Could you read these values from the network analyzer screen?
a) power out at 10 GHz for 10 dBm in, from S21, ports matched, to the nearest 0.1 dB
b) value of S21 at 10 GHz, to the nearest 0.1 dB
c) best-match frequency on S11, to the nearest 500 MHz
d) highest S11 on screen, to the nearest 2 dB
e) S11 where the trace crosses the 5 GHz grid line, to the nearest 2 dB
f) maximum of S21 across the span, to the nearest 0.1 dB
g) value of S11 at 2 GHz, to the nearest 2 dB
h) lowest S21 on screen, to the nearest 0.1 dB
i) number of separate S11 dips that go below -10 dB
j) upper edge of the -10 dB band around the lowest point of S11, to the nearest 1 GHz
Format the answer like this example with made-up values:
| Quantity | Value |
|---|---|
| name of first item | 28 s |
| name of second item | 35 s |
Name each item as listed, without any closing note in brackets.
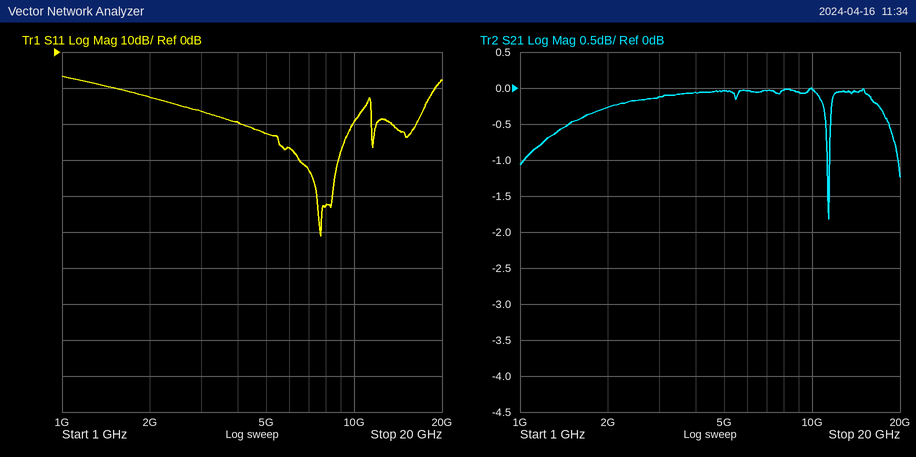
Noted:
| Quantity | Value |
|---|---|
| power out at 10 GHz for 10 dBm in, from S21, ports matched, to the nearest 0.1 dB | 10.0 dBm |
| value of S21 at 10 GHz, to the nearest 0.1 dB | 0.0 dB |
| best-match frequency on S11, to the nearest 500 MHz | 7.5 GHz |
| highest S11 on screen, to the nearest 2 dB | -6 dB |
| S11 where the trace crosses the 5 GHz grid line, to the nearest 2 dB | -22 dB |
| maximum of S21 across the span, to the nearest 0.1 dB | 0.0 dB |
| value of S11 at 2 GHz, to the nearest 2 dB | -12 dB |
| lowest S21 on screen, to the nearest 0.1 dB | -1.8 dB |
| number of separate S11 dips that go below -10 dB | 3 |
| upper edge of the -10 dB band around the lowest point of S11, to the nearest 1 GHz | 19 GHz |
